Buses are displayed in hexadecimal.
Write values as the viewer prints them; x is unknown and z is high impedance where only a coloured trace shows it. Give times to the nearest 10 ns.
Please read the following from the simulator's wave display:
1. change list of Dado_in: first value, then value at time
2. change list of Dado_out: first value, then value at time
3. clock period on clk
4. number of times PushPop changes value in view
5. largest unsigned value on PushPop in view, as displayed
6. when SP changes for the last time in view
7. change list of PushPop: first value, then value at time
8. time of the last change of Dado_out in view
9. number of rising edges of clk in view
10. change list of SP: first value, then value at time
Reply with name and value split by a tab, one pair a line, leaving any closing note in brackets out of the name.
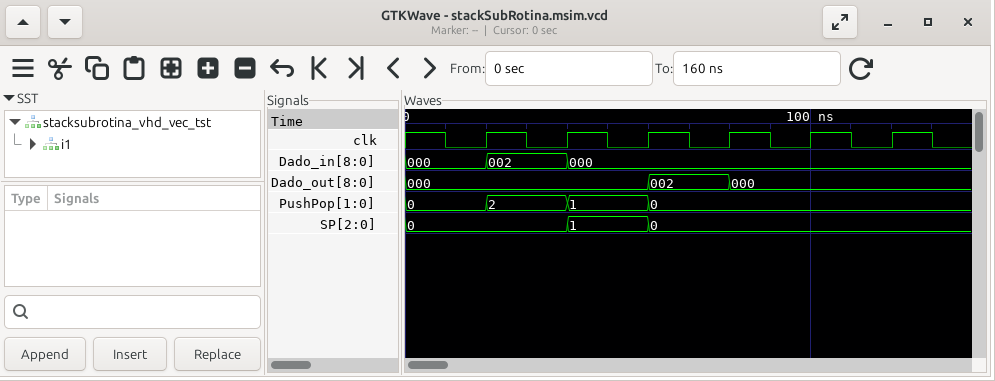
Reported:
change list of Dado_in: first value, then value at time	000, 002 at 20 ns, 000 at 40 ns
change list of Dado_out: first value, then value at time	000, 002 at 60 ns, 000 at 80 ns
clock period on clk	20 ns
number of times PushPop changes value in view	3
largest unsigned value on PushPop in view, as displayed	2
when SP changes for the last time in view	60 ns
change list of PushPop: first value, then value at time	0, 2 at 20 ns, 1 at 40 ns, 0 at 60 ns
time of the last change of Dado_out in view	80 ns
number of rising edges of clk in view	6
change list of SP: first value, then value at time	0, 1 at 40 ns, 0 at 60 ns
